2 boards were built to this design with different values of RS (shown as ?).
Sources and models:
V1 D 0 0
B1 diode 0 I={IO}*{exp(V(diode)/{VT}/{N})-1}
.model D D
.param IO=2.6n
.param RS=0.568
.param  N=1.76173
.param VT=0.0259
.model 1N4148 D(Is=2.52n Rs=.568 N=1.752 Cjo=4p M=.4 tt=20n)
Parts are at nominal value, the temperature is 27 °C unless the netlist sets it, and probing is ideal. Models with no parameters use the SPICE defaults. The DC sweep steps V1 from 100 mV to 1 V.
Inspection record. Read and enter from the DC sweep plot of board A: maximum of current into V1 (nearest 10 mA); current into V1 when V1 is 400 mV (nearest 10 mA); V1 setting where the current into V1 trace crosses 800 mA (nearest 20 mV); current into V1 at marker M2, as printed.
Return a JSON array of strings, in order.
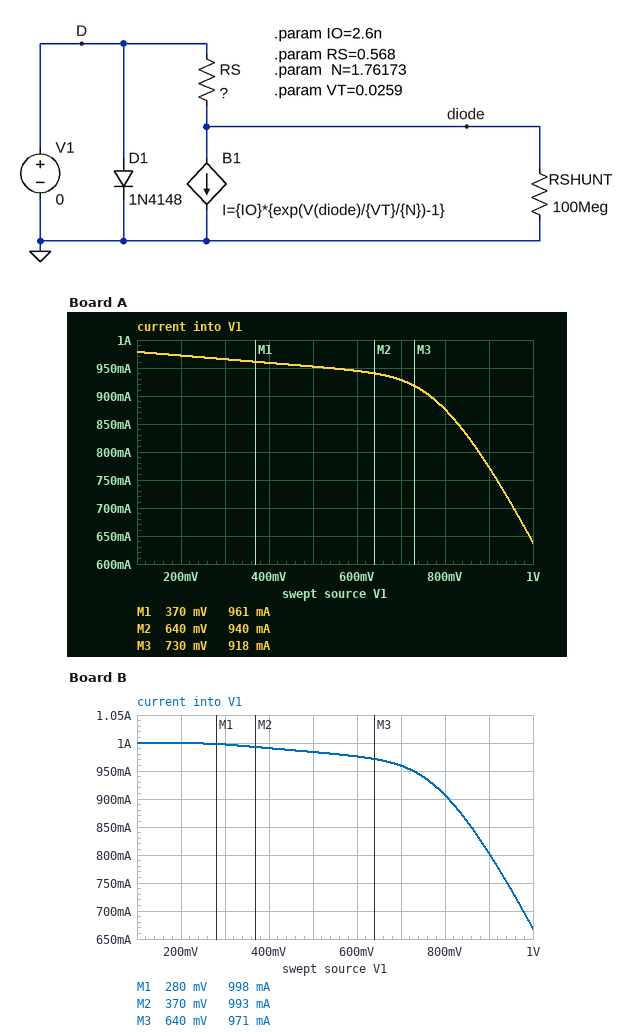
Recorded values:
["980 mA", "960 mA", "880 mV", "940 mA"]
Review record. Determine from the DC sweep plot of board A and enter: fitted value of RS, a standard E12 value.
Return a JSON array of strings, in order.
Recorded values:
["0.82 Ω"]
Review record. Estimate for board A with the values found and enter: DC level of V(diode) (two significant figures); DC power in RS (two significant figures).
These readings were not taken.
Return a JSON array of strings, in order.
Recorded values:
["810 mV", "800 mW"]
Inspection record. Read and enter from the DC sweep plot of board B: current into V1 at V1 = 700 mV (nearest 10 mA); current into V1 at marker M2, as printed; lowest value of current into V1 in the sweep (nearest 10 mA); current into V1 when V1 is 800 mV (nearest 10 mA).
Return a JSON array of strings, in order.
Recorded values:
["960 mA", "993 mA", "670 mA", "910 mA"]
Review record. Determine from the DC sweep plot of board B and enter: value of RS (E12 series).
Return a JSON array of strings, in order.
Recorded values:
["0.33 Ω"]
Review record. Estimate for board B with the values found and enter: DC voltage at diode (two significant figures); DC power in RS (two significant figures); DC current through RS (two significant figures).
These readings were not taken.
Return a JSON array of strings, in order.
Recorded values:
["330 mV", "330 mW", "1.0 A"]
